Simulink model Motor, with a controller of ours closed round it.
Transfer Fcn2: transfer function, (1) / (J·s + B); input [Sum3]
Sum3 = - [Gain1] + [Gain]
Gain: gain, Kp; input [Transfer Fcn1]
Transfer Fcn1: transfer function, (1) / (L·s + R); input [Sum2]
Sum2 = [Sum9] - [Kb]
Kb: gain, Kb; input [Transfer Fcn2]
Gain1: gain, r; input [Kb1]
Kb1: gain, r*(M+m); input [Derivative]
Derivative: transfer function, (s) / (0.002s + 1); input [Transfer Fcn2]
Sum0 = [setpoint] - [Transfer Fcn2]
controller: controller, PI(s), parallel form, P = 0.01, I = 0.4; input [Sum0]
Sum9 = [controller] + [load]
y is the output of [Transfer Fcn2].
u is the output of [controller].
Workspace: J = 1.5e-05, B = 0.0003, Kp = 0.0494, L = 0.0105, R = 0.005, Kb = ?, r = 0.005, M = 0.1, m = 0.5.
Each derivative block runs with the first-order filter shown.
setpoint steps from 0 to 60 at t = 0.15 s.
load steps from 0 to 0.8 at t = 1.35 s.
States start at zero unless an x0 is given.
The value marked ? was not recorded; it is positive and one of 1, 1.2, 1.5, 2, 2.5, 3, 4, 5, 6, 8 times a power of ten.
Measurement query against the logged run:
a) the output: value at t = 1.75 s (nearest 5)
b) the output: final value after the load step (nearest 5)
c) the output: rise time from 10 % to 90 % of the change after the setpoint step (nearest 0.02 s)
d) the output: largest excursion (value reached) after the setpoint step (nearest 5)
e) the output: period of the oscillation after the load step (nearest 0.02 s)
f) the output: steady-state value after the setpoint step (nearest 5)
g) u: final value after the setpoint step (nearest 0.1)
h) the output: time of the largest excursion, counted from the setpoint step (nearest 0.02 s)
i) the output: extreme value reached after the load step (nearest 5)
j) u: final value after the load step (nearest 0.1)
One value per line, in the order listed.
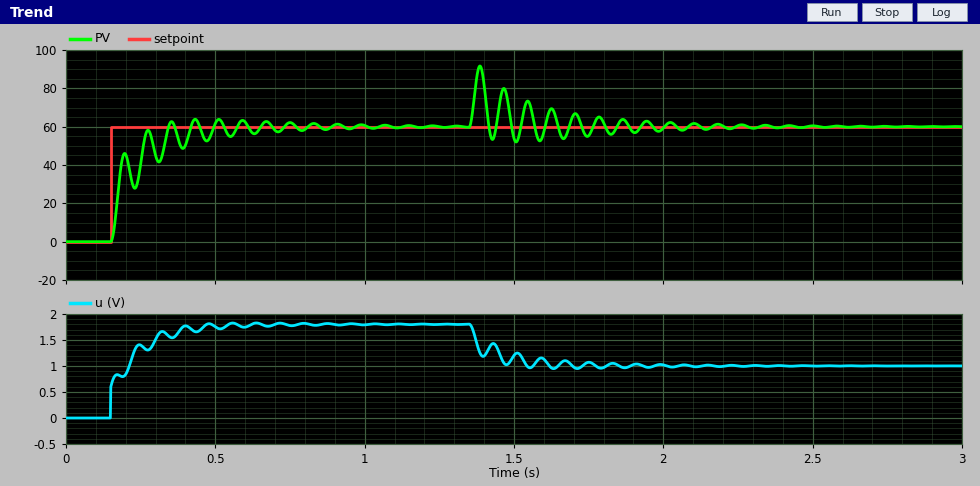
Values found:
55
60
0.10 s
65
0.08 s
60
1.8
0.28 s
90
1.0
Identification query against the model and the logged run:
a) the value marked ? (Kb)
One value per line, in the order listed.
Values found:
0.03
